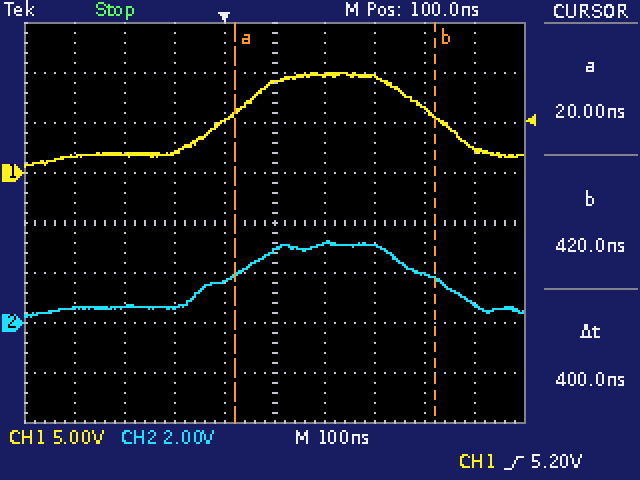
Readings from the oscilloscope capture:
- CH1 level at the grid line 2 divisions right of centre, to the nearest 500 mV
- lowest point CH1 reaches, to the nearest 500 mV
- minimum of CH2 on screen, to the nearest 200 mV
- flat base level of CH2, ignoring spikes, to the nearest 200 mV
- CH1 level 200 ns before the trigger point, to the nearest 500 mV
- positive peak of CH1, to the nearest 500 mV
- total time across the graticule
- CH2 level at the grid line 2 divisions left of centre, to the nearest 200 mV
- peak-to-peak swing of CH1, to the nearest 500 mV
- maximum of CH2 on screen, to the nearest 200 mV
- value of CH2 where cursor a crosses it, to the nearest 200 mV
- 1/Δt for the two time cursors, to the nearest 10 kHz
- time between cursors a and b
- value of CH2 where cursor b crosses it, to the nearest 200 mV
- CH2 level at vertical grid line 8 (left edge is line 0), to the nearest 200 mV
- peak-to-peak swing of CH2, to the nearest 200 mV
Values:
9.5 V
500 mV
200 mV
600 mV
2.0 V
10.0 V
1 µs
600 mV
9.5 V
3.2 V
2.0 V
2.50 MHz
400 ns
1.8 V
2.0 V
3.0 V
